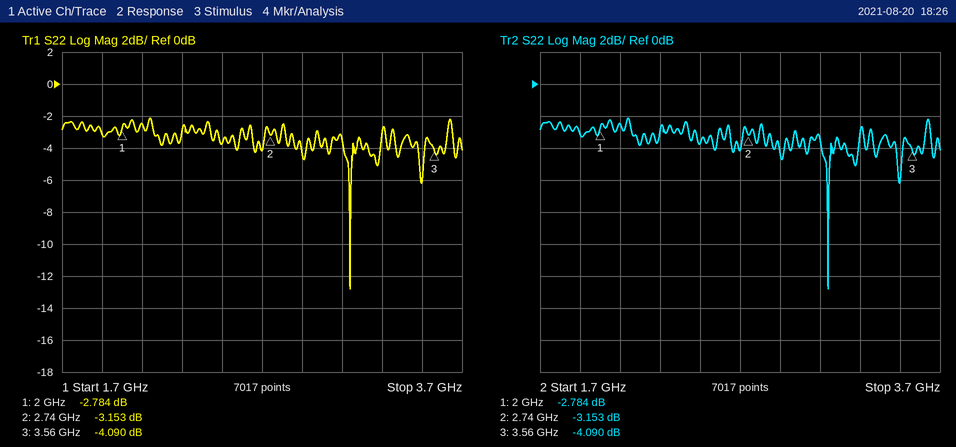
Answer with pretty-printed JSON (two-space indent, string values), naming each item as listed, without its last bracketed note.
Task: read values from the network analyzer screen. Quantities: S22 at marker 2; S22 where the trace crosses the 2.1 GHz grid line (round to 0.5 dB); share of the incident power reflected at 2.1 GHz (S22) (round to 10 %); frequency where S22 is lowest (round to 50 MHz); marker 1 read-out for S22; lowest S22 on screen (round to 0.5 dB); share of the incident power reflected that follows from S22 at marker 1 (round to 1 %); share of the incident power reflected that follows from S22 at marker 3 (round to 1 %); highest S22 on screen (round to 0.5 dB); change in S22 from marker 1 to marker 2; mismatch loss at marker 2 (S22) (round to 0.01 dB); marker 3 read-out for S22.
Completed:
{
  "S22 at marker 2": "-3.153 dB",
  "S22 where the trace crosses the 2.1 GHz grid line": "-2.5 dB",
  "share of the incident power reflected at 2.1 GHz (S22)": "60 %",
  "frequency where S22 is lowest": "3.15 GHz",
  "marker 1 read-out for S22": "-2.784 dB",
  "lowest S22 on screen": "-13.0 dB",
  "share of the incident power reflected that follows from S22 at marker 1": "53 %",
  "share of the incident power reflected that follows from S22 at marker 3": "39 %",
  "highest S22 on screen": "-2.0 dB",
  "change in S22 from marker 1 to marker 2": "-0.369 dB",
  "mismatch loss at marker 2 (S22)": "2.87 dB",
  "marker 3 read-out for S22": "-4.090 dB"
}
